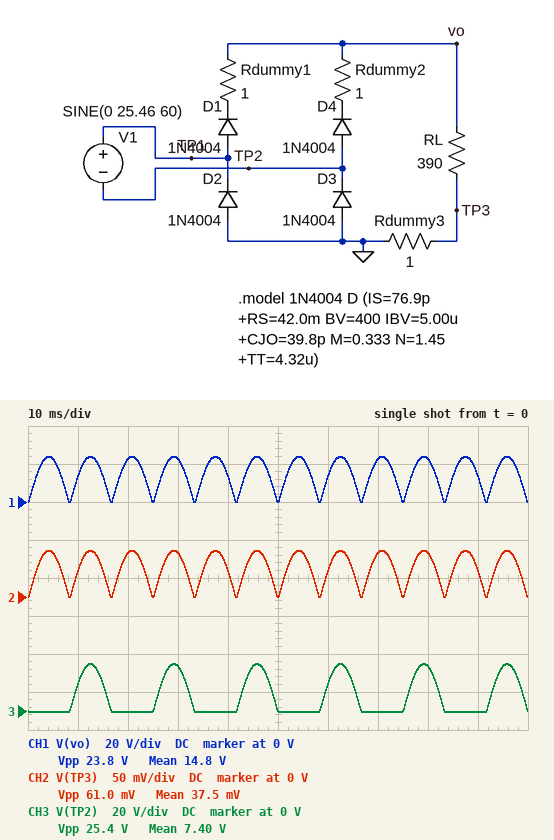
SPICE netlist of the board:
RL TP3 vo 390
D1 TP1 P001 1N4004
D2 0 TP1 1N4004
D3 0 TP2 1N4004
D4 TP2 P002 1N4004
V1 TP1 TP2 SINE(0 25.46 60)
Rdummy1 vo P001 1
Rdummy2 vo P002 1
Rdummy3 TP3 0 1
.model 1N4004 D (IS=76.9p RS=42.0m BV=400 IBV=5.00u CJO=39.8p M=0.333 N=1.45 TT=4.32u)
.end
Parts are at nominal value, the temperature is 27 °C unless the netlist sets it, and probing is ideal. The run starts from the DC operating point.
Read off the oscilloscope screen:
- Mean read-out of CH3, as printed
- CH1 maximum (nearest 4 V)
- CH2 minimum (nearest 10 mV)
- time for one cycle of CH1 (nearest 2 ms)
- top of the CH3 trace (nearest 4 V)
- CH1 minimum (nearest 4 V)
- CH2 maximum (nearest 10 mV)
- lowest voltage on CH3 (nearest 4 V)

7.40 V
24 V
0 V
8 ms
24 V
0 V
60 mV
0 V
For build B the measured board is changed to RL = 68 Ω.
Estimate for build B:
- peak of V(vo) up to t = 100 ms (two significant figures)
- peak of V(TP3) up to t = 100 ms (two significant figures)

23 V
340 mV
